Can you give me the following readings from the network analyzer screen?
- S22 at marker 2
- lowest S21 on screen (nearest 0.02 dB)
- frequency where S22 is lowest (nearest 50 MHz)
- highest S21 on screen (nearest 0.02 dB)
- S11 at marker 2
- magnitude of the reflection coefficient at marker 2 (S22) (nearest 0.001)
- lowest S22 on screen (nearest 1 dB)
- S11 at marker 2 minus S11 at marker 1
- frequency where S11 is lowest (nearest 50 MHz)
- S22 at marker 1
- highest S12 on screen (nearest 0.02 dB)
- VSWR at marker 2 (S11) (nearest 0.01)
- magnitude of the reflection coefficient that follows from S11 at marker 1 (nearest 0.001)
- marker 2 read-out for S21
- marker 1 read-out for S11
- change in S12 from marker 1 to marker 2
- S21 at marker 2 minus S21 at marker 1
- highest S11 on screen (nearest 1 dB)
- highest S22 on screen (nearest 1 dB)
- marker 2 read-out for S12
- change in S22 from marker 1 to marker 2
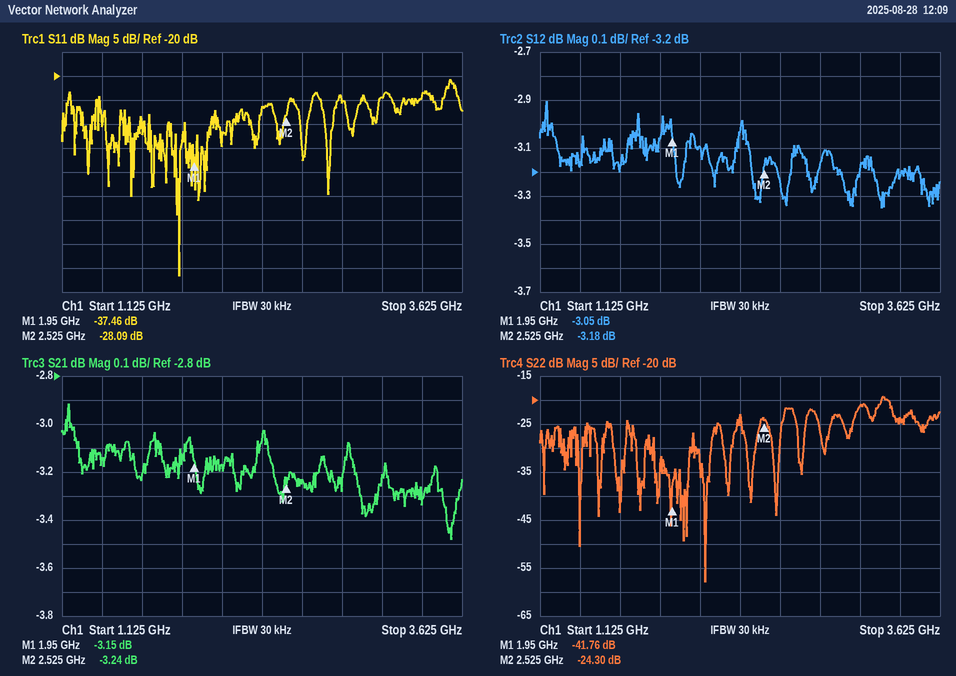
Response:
-24.30 dB
-3.48 dB
2.15 GHz
-2.92 dB
-28.09 dB
0.061
-58 dB
9.37 dB
1.85 GHz
-41.76 dB
-2.90 dB
1.08
0.013
-3.24 dB
-37.46 dB
-0.13 dB
-0.09 dB
-21 dB
-19 dB
-3.18 dB
17.46 dB
